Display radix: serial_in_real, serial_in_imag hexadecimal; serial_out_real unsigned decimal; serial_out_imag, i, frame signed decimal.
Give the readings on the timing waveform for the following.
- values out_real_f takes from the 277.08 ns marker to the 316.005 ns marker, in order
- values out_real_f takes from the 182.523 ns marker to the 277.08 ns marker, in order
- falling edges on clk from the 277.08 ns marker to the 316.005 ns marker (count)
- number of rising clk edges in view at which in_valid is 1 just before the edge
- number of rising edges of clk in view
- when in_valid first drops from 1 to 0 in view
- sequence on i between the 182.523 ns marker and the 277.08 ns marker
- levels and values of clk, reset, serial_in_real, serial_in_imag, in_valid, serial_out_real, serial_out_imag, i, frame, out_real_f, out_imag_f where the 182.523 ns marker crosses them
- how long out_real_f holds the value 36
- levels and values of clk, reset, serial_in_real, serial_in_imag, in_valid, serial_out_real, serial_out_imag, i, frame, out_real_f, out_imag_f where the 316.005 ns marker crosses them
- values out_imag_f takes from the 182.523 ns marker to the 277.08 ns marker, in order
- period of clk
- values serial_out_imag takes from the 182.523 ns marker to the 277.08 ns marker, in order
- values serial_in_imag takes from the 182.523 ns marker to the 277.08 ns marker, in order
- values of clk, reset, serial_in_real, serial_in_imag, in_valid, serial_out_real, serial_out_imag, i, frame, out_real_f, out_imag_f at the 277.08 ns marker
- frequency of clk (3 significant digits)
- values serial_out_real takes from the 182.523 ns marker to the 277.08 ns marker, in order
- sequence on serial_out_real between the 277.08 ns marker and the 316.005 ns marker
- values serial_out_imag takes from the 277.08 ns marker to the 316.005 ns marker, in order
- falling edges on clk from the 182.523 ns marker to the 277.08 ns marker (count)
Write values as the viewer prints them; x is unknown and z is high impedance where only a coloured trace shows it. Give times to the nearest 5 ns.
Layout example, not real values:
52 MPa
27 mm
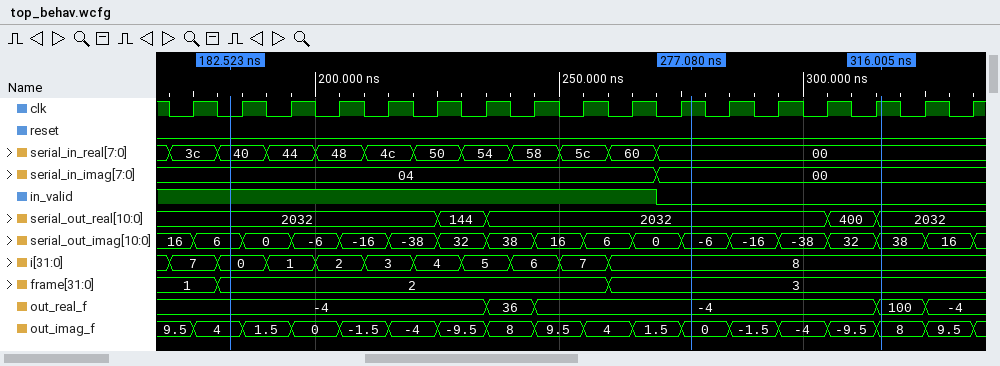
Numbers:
-4, 100
-4, 36, -4
4
10
17
270 ns
0, 1, 2, 3, 4, 5, 6, 7, 8
clk=0, reset=0, serial_in_real=40, serial_in_imag=04, in_valid=1, serial_out_real=2032, serial_out_imag=6, i=0, frame=2, out_real_f=-4, out_imag_f=4
10 ns
clk=1, reset=0, serial_in_real=00, serial_in_imag=00, in_valid=0, serial_out_real=2032, serial_out_imag=38, i=8, frame=3, out_real_f=100, out_imag_f=8
4, 1.5, 0, -1.5, -4, -9.5, 8, 9.5, 4, 1.5, 0
10 ns
6, 0, -6, -16, -38, 32, 38, 16, 6, 0, -6
04, 00
clk=1, reset=0, serial_in_real=00, serial_in_imag=00, in_valid=0, serial_out_real=2032, serial_out_imag=-6, i=8, frame=3, out_real_f=-4, out_imag_f=0
100 MHz
2032, 144, 2032
2032, 400, 2032
-6, -16, -38, 32, 38
9
